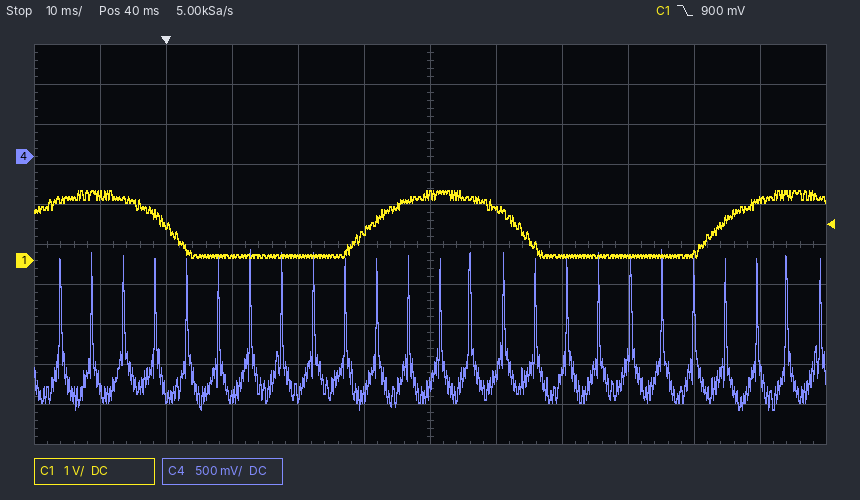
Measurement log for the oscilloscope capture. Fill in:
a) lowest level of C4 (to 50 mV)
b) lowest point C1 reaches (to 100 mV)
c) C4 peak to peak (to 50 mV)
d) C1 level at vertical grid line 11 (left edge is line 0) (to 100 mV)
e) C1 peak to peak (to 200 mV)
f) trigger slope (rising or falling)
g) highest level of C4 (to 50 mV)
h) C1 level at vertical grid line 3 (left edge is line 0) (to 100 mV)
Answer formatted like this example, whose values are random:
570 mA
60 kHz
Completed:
-3.15 V
100 mV
2.00 V
1.5 V
1.6 V
falling
-1.15 V
100 mV
